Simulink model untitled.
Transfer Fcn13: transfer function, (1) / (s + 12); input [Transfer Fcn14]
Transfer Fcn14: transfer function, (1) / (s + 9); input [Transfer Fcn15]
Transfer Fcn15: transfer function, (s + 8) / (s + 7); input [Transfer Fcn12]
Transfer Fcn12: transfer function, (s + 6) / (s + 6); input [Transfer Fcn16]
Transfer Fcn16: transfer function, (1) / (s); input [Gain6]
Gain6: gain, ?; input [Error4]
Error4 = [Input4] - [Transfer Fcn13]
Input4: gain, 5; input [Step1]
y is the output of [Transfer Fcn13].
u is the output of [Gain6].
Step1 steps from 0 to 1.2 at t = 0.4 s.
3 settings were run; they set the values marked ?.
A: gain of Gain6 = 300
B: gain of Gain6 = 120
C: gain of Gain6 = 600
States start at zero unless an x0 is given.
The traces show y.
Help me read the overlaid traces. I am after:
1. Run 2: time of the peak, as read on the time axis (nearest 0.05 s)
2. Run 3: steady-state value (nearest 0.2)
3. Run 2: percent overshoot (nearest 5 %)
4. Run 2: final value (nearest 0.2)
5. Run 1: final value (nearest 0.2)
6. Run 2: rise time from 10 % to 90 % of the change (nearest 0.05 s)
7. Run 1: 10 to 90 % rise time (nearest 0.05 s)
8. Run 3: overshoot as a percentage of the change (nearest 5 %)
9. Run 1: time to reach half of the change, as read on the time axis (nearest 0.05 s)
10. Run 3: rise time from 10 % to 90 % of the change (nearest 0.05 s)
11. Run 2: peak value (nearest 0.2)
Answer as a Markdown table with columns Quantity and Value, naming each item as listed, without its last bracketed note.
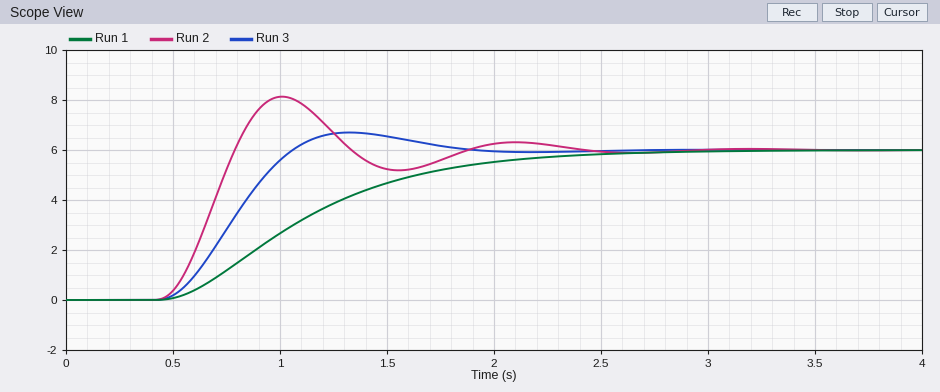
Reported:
| Quantity | Value |
|---|---|
| Run 2: time of the peak, as read on the time axis | 1.00 s |
| Run 3: steady-state value | 6.0 |
| Run 2: percent overshoot | 35 % |
| Run 2: final value | 6.0 |
| Run 1: final value | 6.0 |
| Run 2: rise time from 10 % to 90 % of the change | 0.25 s |
| Run 1: 10 to 90 % rise time | 1.25 s |
| Run 3: overshoot as a percentage of the change | 10 % |
| Run 1: time to reach half of the change, as read on the time axis | 1.05 s |
| Run 3: rise time from 10 % to 90 % of the change | 0.40 s |
| Run 2: peak value | 8.2 |
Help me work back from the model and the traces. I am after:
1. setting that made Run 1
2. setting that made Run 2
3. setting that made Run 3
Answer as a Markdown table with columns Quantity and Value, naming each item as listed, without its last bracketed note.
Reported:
| Quantity | Value |
|---|---|
| setting that made Run 1 | B |
| setting that made Run 2 | C |
| setting that made Run 3 | A |
